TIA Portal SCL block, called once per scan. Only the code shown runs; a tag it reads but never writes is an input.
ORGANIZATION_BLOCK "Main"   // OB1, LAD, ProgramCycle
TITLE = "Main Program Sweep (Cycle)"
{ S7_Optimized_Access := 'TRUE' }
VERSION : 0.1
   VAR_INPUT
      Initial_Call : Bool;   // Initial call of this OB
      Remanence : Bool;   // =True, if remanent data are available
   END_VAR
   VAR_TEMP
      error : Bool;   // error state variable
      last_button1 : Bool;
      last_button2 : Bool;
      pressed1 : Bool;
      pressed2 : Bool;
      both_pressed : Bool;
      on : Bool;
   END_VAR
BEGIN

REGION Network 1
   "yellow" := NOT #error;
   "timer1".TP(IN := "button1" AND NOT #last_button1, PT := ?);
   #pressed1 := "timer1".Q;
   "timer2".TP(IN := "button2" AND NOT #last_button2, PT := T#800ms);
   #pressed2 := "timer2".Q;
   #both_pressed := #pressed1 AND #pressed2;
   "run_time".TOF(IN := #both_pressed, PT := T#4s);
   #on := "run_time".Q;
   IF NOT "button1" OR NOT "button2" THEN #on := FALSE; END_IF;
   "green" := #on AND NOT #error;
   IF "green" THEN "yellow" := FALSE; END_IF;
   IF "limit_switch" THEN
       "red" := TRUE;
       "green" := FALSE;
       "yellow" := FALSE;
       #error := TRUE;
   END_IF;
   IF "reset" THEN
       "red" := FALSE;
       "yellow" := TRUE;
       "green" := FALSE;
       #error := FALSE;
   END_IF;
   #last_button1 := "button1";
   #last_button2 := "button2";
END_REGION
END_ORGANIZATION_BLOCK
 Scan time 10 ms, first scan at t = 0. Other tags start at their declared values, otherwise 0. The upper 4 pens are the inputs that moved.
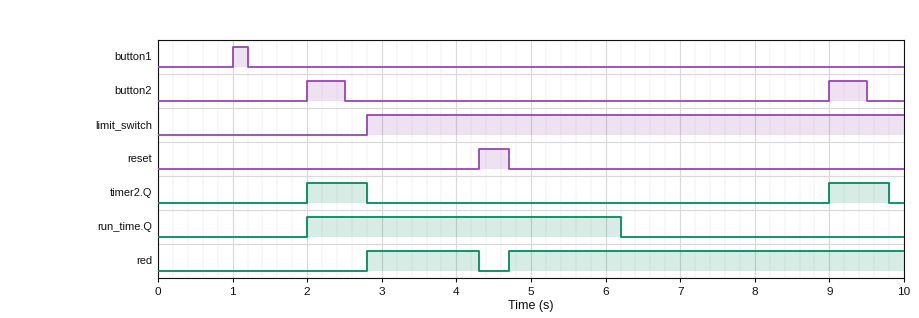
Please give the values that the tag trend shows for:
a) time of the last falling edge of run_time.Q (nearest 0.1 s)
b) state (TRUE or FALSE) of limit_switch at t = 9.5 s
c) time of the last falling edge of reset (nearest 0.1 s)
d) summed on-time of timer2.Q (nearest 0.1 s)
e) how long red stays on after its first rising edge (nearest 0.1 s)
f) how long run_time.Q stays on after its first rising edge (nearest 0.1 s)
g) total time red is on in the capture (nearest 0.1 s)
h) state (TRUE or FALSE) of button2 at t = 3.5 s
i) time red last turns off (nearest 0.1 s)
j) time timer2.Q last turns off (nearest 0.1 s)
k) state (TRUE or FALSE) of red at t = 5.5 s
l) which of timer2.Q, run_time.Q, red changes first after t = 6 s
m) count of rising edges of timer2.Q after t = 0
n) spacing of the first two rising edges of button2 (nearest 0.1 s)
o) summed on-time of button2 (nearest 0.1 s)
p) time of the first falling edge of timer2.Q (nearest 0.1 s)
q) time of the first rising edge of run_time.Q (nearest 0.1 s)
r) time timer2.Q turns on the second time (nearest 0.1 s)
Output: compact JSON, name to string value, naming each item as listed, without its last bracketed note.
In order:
{"time of the last falling edge of run_time.Q": "6.2 s", "state (TRUE or FALSE) of limit_switch at t = 9.5 s": "TRUE", "time of the last falling edge of reset": "4.7 s", "summed on-time of timer2.Q": "1.6 s", "how long red stays on after its first rising edge": "1.5 s", "how long run_time.Q stays on after its first rising edge": "4.2 s", "total time red is on in the capture": "6.8 s", "state (TRUE or FALSE) of button2 at t = 3.5 s": "FALSE", "time red last turns off": "4.3 s", "time timer2.Q last turns off": "9.8 s", "state (TRUE or FALSE) of red at t = 5.5 s": "TRUE", "which of timer2.Q, run_time.Q, red changes first after t = 6 s": "run_time.Q", "count of rising edges of timer2.Q after t = 0": "2", "spacing of the first two rising edges of button2": "7.0 s", "summed on-time of button2": "1.0 s", "time of the first falling edge of timer2.Q": "2.8 s", "time of the first rising edge of run_time.Q": "2.0 s", "time timer2.Q turns on the second time": "9.0 s"}
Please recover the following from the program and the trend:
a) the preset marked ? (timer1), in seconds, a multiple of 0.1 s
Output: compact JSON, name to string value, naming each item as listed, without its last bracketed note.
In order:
{"the preset marked ? (timer1), in seconds, a multiple of 0.1 s": "1.2 s"}
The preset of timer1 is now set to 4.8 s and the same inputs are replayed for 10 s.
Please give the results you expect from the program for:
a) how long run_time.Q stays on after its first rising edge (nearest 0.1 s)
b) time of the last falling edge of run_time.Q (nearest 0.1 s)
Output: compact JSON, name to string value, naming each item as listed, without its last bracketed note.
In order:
{"how long run_time.Q stays on after its first rising edge": "4.8 s", "time of the last falling edge of run_time.Q": "6.8 s"}
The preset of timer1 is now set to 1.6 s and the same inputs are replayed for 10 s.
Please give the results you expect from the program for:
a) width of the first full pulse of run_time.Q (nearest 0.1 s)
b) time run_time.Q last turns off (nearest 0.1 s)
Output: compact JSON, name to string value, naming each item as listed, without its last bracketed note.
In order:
{"width of the first full pulse of run_time.Q": "4.6 s", "time run_time.Q last turns off": "6.6 s"}
